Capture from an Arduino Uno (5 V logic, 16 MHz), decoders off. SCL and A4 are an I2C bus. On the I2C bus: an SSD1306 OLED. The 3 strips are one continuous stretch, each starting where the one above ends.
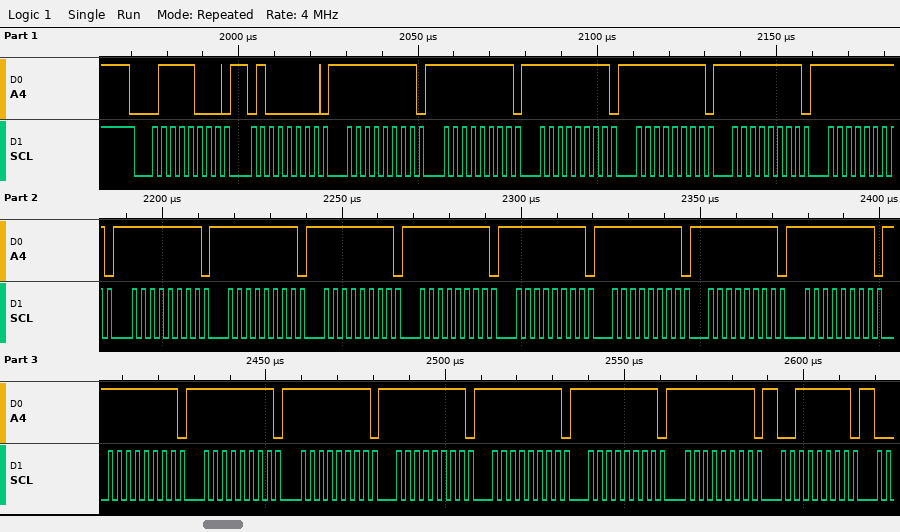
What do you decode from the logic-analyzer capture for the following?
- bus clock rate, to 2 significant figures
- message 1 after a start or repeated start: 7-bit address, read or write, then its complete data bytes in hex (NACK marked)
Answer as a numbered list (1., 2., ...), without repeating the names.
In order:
1. 400 kHz
2. 0x3C write: 40 FF FF FF FF FF FF FF FF FF FF FF FF FF FF FF FF FF FF FF FF FF 3F
